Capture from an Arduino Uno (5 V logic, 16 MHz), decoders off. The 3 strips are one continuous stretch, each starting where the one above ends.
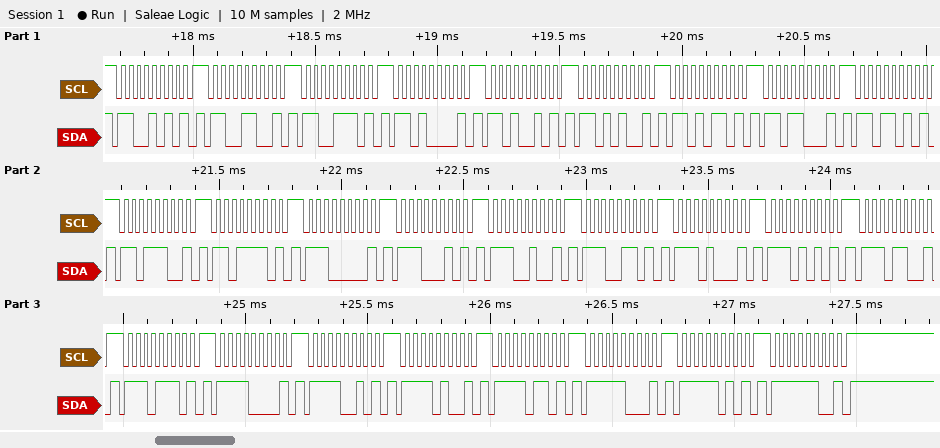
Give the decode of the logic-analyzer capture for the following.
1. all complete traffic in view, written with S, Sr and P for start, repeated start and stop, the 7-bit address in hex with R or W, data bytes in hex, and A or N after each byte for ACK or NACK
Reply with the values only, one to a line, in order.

S 65W N P S 66W N P S 67W N P S 68W N P S 69W N P S 6AW N P S 6BW N P S 6CW N P S 6DW N P S 6EW N P S 6FW N P S 70W N P S 71W N P S 72W N P S 73W N P S 74W N P S 75W N P S 76W N P S 77W N P S 78W N P S 79W N P S 7AW N P S 7BW N P S 7CW N P S 7DW N P S 7EW N P
